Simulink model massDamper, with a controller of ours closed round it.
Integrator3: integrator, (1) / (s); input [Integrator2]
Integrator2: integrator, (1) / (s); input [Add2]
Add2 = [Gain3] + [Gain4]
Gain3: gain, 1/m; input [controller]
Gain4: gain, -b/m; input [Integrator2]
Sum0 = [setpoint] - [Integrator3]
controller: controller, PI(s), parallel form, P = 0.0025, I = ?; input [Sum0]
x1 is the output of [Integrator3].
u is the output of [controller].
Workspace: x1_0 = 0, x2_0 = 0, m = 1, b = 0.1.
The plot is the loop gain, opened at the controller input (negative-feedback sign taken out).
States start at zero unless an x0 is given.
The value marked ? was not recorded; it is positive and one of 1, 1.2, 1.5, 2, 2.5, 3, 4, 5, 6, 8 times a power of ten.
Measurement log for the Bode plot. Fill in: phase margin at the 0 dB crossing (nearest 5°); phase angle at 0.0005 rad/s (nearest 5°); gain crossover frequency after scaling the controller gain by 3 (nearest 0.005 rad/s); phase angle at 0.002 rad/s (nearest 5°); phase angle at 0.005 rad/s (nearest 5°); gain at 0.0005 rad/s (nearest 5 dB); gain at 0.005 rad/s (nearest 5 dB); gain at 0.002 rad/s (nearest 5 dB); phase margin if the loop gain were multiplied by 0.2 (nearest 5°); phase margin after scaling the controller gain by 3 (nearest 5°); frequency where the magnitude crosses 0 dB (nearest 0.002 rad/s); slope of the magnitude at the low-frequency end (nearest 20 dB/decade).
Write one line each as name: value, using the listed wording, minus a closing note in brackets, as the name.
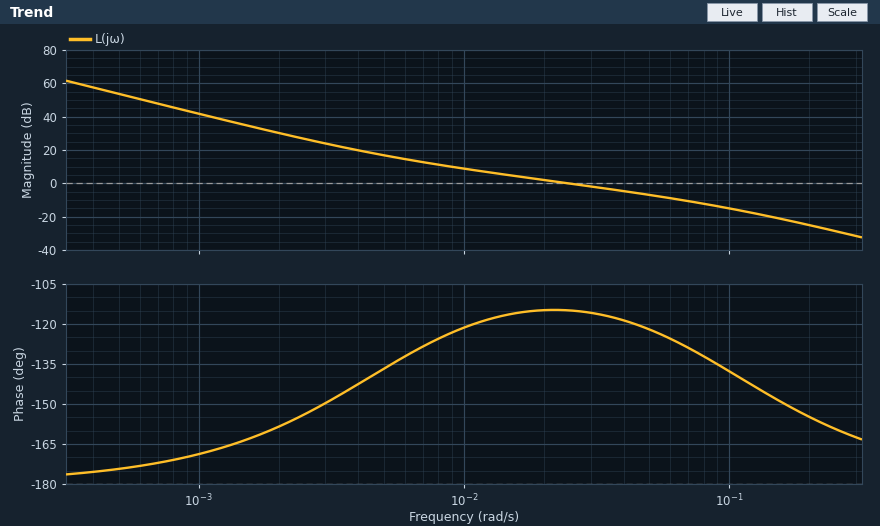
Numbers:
phase margin at the 0 dB crossing: 65°
phase angle at 0.0005 rad/s: -175°
gain crossover frequency after scaling the controller gain by 3: 0.065 rad/s
phase angle at 0.002 rad/s: -160°
phase angle at 0.005 rad/s: -135°
gain at 0.0005 rad/s: 55 dB
gain at 0.005 rad/s: 15 dB
gain at 0.002 rad/s: 30 dB
phase margin if the loop gain were multiplied by 0.2: 50°
phase margin after scaling the controller gain by 3: 55°
frequency where the magnitude crosses 0 dB: 0.024 rad/s
slope of the magnitude at the low-frequency end: -40 dB/decade
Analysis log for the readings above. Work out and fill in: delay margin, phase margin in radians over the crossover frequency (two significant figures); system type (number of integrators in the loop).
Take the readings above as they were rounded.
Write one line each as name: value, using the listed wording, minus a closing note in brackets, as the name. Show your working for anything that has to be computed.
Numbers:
delay margin, phase margin in radians over the crossover frequency: 65 × π / 180 / 0.024 = 47 s
system type: 2
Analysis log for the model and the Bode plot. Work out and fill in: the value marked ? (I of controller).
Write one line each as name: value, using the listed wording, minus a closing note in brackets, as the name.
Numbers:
the value marked ?: 1.2e-05
